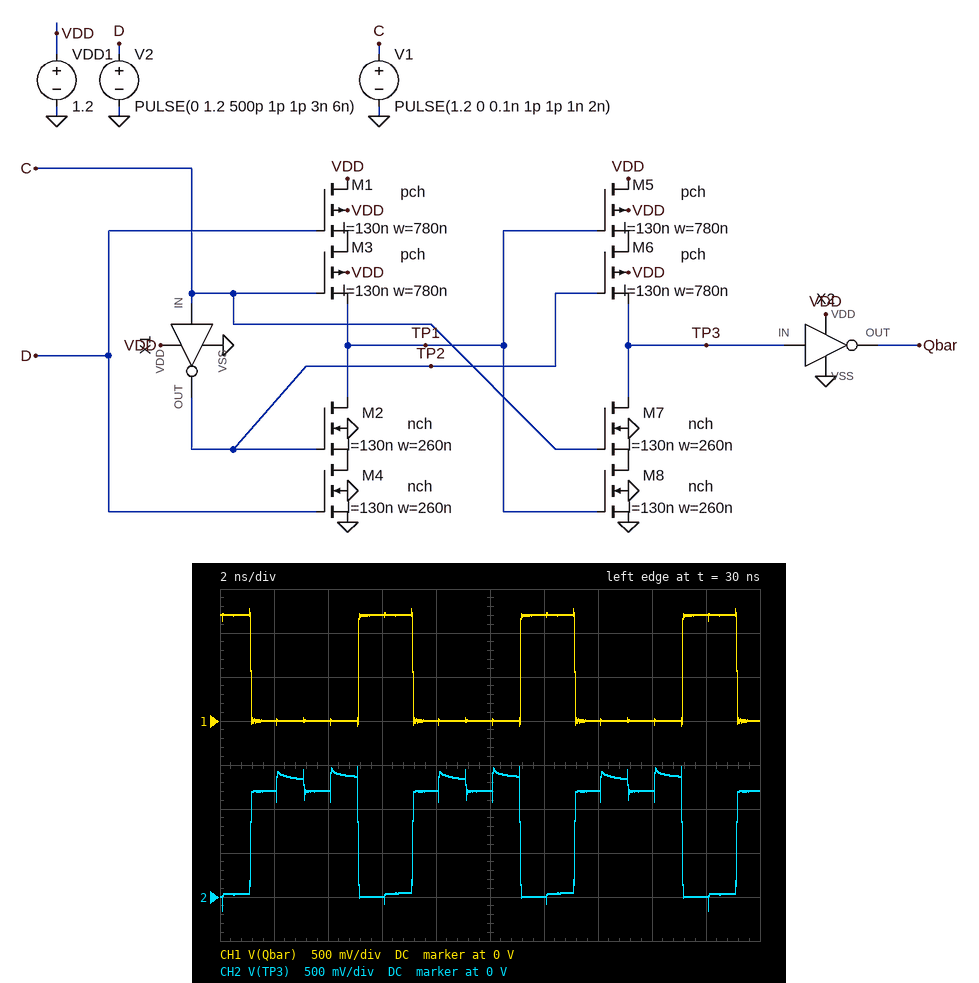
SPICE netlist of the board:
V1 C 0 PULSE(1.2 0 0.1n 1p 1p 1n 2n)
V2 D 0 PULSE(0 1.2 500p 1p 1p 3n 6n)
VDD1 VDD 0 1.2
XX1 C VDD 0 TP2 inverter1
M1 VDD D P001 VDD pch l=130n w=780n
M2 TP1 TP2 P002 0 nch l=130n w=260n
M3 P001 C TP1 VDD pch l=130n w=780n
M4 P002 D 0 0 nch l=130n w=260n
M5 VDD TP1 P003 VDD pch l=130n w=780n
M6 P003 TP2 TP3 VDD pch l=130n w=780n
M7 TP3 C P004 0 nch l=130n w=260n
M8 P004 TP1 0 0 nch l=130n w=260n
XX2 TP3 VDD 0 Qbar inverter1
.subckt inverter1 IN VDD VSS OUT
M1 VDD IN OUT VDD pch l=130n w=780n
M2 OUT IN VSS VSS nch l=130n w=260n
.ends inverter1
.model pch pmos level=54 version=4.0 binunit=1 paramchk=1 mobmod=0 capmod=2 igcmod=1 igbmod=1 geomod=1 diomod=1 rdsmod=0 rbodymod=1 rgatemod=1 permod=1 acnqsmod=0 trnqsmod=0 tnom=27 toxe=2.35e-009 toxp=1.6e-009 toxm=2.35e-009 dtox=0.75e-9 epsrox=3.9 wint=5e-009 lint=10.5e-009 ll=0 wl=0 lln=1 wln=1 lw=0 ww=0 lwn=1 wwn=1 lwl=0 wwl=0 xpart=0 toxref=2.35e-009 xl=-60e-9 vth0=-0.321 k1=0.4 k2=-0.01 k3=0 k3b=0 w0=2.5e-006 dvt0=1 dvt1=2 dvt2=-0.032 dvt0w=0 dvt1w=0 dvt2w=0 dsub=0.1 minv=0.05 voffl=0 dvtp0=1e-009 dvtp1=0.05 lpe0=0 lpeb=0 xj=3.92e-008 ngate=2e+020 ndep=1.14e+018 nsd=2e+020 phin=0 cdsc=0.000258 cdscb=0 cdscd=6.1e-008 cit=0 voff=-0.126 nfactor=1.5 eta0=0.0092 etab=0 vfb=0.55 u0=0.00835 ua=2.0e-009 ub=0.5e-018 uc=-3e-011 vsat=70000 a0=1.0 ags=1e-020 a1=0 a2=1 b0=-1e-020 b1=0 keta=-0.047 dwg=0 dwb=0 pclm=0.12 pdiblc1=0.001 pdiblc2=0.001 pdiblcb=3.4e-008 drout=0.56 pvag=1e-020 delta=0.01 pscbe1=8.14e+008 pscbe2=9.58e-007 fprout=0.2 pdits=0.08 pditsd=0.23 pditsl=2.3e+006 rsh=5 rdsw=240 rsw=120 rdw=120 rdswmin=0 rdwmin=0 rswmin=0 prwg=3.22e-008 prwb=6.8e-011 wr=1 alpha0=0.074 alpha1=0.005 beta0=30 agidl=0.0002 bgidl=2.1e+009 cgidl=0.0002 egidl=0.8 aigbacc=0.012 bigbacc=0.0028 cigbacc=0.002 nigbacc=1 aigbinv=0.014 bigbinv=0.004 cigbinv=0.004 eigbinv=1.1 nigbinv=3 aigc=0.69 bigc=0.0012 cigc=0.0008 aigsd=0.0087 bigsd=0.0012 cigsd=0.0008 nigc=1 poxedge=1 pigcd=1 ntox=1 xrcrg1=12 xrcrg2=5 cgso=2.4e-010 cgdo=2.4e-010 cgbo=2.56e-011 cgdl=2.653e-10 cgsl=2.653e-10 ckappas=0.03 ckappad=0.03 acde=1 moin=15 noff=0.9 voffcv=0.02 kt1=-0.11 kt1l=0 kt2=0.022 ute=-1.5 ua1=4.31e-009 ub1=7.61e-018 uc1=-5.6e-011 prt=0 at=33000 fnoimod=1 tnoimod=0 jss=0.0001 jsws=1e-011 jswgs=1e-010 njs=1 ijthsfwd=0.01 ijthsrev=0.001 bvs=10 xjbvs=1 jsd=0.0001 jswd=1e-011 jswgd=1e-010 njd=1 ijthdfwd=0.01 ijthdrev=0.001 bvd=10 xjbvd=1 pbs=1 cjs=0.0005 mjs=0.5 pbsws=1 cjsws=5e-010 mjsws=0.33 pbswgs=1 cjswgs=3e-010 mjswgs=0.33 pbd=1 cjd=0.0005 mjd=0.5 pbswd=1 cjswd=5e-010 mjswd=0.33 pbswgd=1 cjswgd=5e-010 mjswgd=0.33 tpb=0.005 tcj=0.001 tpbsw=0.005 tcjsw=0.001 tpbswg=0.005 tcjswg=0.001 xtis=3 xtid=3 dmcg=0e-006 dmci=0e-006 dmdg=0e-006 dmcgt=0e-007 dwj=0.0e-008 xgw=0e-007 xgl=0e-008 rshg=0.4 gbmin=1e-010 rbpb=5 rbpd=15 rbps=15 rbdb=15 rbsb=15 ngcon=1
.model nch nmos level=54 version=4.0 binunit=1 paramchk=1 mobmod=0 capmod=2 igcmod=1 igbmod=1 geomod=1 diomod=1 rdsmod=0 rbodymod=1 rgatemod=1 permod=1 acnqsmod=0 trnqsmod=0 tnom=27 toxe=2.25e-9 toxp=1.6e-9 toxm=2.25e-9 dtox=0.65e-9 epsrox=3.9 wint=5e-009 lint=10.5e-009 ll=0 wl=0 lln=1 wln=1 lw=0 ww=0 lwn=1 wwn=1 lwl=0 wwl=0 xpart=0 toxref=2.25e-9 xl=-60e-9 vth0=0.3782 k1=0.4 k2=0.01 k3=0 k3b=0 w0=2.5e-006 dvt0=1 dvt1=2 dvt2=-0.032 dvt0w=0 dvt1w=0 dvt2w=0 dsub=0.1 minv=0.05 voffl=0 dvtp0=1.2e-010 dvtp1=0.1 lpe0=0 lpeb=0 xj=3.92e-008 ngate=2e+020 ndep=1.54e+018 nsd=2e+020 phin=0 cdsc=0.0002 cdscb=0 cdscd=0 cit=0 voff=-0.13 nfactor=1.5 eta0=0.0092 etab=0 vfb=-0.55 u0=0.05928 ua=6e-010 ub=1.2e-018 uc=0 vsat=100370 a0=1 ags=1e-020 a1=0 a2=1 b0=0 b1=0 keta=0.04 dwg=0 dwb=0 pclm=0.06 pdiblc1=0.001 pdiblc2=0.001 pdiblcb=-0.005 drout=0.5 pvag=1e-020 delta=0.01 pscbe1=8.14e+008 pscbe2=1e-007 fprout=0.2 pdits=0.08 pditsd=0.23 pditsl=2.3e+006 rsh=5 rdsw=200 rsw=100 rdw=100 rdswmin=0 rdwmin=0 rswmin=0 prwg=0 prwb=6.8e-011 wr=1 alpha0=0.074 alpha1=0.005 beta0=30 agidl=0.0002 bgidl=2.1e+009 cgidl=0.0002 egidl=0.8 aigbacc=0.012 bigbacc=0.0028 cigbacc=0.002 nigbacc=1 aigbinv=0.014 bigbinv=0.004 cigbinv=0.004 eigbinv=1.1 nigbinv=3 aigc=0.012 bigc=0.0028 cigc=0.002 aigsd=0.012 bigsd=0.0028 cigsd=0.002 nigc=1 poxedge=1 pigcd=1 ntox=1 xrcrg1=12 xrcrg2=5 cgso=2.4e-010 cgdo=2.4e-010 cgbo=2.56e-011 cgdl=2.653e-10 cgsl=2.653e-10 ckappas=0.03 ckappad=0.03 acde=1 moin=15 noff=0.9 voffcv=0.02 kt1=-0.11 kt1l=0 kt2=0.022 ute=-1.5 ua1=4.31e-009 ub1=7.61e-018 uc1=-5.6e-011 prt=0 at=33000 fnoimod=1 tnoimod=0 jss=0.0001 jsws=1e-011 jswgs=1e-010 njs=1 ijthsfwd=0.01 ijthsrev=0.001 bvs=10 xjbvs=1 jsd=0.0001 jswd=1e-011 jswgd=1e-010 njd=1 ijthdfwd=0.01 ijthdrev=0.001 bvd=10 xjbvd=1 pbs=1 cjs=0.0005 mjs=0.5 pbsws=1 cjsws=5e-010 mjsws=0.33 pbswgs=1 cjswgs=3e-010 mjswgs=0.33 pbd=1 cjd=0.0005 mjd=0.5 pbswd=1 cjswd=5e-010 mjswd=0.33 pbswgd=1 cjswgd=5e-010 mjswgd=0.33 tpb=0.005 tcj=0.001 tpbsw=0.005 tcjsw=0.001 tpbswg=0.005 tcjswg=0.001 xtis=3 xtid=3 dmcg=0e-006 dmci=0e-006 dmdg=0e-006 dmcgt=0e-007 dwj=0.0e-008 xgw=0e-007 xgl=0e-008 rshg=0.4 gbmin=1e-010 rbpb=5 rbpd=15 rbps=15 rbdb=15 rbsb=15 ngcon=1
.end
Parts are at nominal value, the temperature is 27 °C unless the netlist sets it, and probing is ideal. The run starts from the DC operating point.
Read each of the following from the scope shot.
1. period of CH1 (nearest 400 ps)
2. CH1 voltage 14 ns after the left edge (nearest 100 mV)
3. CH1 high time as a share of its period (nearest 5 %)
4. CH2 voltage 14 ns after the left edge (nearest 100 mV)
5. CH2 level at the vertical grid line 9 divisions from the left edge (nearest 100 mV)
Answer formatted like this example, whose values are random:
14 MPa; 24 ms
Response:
6.0 ns; 0 V; 35 %; 1.2 V; 0 V
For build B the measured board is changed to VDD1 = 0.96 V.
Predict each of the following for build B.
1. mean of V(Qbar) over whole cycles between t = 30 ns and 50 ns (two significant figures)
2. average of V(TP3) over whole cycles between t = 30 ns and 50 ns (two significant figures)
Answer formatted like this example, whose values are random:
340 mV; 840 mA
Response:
320 mV; 690 mV
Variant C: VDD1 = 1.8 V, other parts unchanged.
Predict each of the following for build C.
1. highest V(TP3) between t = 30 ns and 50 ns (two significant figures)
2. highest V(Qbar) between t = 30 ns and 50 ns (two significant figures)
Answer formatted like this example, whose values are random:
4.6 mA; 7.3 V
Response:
1.7 V; 1.9 V
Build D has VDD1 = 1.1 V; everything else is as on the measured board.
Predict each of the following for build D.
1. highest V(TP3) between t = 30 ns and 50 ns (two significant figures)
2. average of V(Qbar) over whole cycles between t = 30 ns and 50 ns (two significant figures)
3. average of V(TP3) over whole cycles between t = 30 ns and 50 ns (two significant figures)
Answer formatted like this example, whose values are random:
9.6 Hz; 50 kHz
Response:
1.4 V; 370 mV; 790 mV
